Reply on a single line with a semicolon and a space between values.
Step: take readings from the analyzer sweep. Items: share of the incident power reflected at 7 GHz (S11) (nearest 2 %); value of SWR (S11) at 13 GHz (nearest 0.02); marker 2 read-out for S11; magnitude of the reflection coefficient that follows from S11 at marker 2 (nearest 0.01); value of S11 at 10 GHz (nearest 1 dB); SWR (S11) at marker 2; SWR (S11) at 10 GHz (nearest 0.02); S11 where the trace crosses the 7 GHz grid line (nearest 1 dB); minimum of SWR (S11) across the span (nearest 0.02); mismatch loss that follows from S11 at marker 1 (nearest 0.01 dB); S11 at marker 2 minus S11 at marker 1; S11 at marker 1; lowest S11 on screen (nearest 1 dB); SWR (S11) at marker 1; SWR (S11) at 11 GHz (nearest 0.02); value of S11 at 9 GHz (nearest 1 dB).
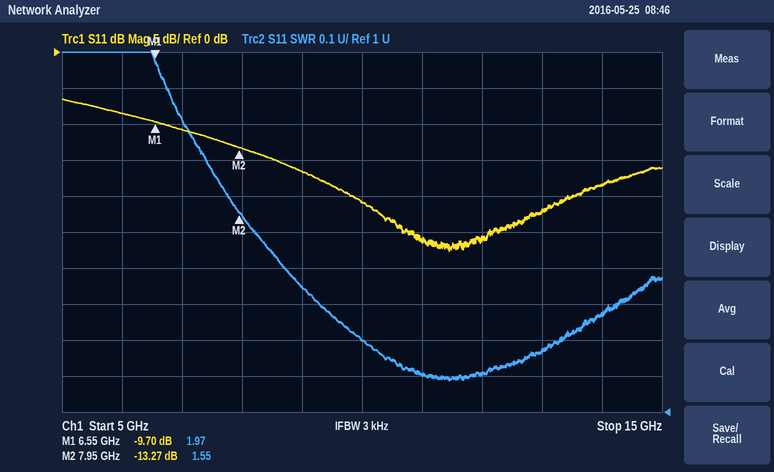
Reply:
8 %; 1.16; -13.27 dB; 0.22; -21 dB; 1.55; 1.20; -11 dB; 1.08; 0.49 dB; -3.57 dB; -9.70 dB; -28 dB; 1.97; 1.10; -17 dB
